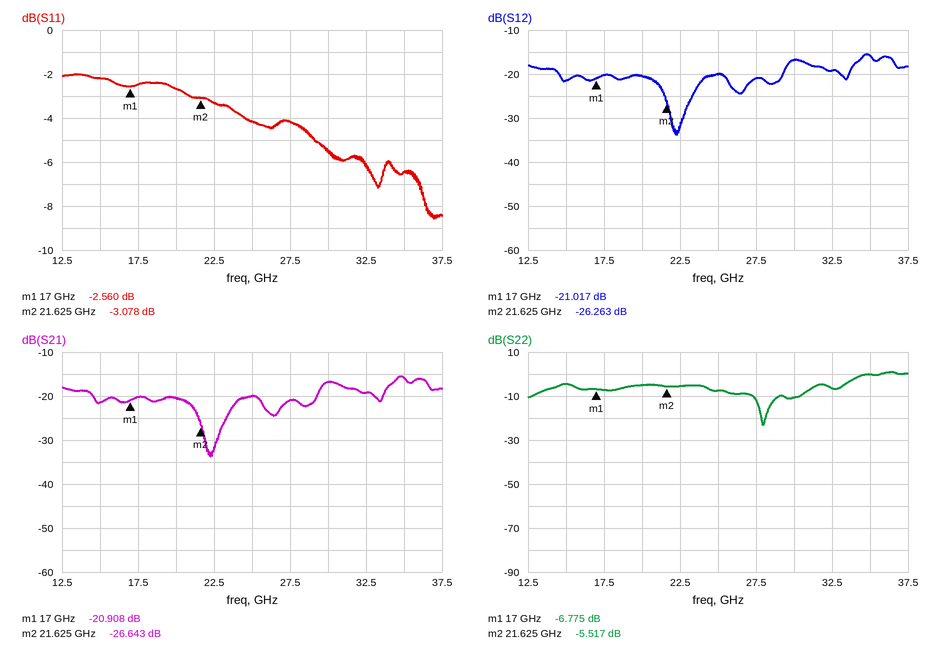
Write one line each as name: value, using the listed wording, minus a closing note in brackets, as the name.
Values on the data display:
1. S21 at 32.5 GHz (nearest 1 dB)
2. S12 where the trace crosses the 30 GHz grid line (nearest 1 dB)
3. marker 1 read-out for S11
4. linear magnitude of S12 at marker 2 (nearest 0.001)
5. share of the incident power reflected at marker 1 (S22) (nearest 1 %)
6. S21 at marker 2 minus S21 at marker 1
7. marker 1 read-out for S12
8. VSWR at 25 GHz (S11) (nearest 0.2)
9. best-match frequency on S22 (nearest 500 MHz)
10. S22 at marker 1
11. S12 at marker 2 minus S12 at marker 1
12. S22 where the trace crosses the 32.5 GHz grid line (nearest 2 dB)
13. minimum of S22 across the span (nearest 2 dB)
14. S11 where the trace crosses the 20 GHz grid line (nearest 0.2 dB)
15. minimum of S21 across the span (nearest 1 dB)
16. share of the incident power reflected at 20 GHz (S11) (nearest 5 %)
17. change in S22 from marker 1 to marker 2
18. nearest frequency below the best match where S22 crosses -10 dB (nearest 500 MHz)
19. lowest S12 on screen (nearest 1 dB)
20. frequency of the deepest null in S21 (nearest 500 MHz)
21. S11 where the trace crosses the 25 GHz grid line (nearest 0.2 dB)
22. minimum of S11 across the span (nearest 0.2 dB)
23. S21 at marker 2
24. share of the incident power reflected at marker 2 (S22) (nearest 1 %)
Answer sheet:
S21 at 32.5 GHz: -19 dB
S12 where the trace crosses the 30 GHz grid line: -17 dB
marker 1 read-out for S11: -2.560 dB
linear magnitude of S12 at marker 2: 0.049
share of the incident power reflected at marker 1 (S22): 21 %
S21 at marker 2 minus S21 at marker 1: -5.735 dB
marker 1 read-out for S12: -21.017 dB
VSWR at 25 GHz (S11): 4.2
best-match frequency on S22: 28.0 GHz
S22 at marker 1: -6.775 dB
S12 at marker 2 minus S12 at marker 1: -5.246 dB
S22 where the trace crosses the 32.5 GHz grid line: -6 dB
minimum of S22 across the span: -24 dB
S11 where the trace crosses the 20 GHz grid line: -2.6 dB
minimum of S21 across the span: -34 dB
share of the incident power reflected at 20 GHz (S11): 55 %
change in S22 from marker 1 to marker 2: 1.258 dB
nearest frequency below the best match where S22 crosses -10 dB: 27.5 GHz
lowest S12 on screen: -34 dB
frequency of the deepest null in S21: 22.5 GHz
S11 where the trace crosses the 25 GHz grid line: -4.2 dB
minimum of S11 across the span: -8.6 dB
S21 at marker 2: -26.643 dB
share of the incident power reflected at marker 2 (S22): 28 %
